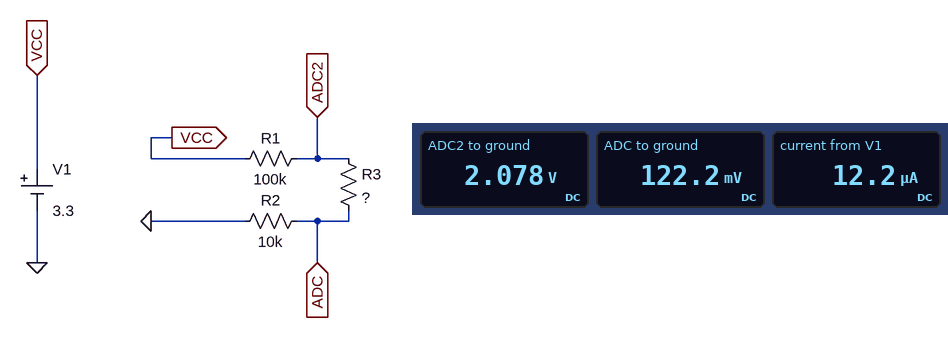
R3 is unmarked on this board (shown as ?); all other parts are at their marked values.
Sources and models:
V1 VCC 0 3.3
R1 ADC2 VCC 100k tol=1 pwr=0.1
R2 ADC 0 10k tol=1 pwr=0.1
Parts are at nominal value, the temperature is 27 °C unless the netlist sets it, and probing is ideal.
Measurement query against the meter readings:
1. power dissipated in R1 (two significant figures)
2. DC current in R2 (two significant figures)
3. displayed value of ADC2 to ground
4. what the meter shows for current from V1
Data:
15 µW
12 µA
2.078 V
12.2 µA
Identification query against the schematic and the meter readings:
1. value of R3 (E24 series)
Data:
160 kΩ
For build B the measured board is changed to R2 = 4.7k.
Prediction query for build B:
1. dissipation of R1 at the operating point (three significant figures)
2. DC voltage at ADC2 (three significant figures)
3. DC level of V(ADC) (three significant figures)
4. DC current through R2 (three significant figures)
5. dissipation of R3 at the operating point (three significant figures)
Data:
15.5 µW
2.05 V
58.6 mV
12.5 µA
24.9 µW
